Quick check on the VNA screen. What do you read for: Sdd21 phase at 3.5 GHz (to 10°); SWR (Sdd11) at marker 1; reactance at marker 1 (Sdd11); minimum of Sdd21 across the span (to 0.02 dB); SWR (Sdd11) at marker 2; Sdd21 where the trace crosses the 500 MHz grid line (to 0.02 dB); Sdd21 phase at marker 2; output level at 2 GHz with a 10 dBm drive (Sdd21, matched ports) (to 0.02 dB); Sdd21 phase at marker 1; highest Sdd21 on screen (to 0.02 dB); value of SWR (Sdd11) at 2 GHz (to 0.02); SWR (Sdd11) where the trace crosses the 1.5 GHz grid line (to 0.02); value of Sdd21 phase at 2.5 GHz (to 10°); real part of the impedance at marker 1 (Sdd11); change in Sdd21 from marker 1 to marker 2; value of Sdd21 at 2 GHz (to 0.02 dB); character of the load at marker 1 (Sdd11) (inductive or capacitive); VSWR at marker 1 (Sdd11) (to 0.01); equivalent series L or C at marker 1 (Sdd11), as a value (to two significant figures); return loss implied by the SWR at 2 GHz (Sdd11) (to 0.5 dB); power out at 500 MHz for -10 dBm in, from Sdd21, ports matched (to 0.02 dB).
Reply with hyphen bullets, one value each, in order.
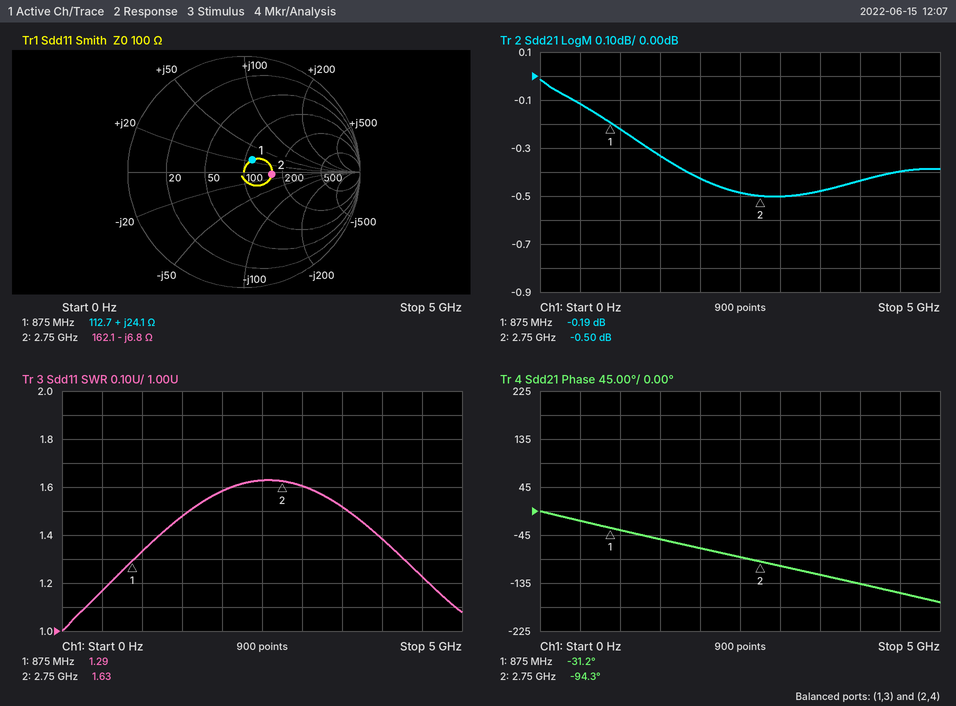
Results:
- -120°
- 1.29
- +24.1 Ω
- -0.50 dB
- 1.63
- -0.12 dB
- -94.3°
- 9.58 dBm
- -31.2°
- -0.02 dB
- 1.58
- 1.48
- -90°
- 112.7 Ω
- -0.31 dB
- -0.42 dB
- inductive
- 1.29
- 4.4 nH
- 13.0 dB
- -10.12 dBm
